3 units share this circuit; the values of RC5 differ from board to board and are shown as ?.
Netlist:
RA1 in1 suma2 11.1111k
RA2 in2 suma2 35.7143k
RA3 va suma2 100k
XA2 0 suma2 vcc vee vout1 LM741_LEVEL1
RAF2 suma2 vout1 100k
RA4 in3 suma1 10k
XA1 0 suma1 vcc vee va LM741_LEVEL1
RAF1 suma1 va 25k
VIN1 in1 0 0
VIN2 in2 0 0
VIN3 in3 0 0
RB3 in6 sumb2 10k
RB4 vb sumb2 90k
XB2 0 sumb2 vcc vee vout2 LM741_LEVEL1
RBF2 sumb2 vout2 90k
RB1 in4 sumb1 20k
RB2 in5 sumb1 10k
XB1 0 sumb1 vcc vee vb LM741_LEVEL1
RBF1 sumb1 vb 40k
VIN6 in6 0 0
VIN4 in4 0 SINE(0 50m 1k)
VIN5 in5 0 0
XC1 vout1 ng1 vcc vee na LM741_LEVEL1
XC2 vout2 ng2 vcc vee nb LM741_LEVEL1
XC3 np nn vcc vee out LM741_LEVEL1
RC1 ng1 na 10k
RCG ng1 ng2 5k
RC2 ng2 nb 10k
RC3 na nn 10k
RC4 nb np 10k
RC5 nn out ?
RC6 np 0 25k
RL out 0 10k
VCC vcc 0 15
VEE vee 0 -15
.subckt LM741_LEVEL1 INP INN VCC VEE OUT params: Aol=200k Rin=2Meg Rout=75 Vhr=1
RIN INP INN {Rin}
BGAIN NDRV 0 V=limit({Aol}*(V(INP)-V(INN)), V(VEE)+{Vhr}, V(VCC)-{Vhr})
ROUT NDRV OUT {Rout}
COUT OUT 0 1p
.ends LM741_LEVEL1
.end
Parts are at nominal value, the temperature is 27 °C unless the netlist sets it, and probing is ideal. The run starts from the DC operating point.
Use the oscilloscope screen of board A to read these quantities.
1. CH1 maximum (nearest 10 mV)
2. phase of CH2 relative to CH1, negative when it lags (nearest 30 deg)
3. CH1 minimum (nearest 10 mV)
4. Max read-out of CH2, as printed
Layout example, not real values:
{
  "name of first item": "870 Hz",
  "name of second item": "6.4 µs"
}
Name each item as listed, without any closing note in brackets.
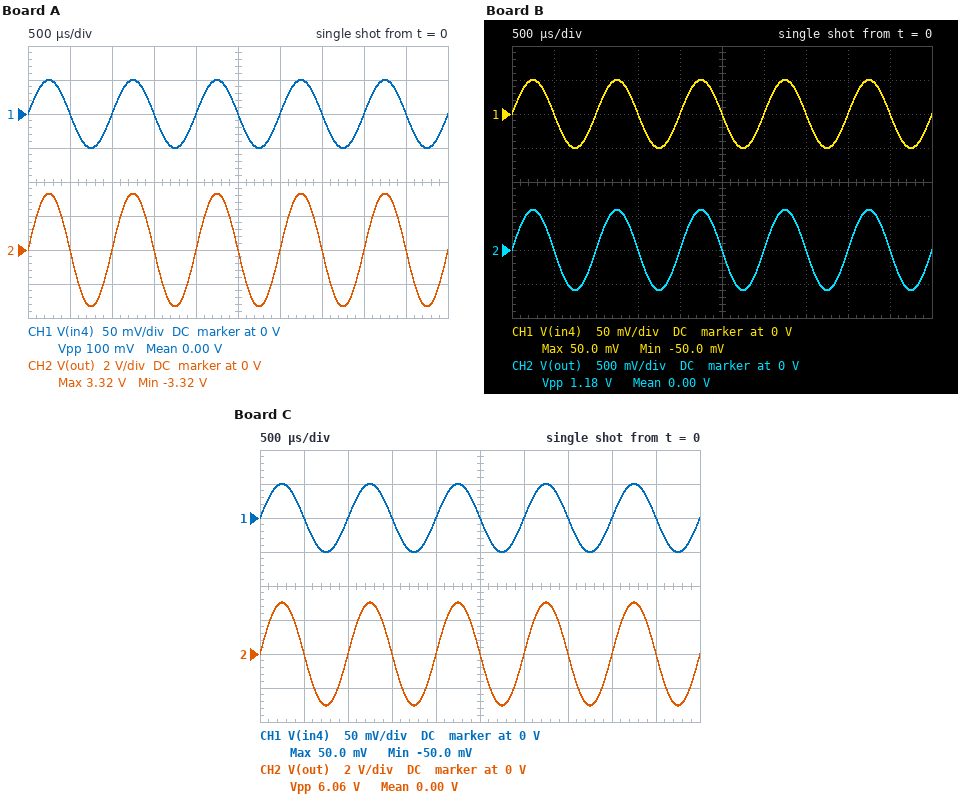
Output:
{
  "CH1 maximum": "50 mV",
  "phase of CH2 relative to CH1, negative when it lags": "0 deg",
  "CH1 minimum": "-50 mV",
  "Max read-out of CH2, as printed": "3.32 V"
}
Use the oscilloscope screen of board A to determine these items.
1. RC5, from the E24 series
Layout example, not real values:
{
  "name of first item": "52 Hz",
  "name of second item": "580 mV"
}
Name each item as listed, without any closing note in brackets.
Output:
{
  "RC5, from the E24 series": "75 kΩ"
}
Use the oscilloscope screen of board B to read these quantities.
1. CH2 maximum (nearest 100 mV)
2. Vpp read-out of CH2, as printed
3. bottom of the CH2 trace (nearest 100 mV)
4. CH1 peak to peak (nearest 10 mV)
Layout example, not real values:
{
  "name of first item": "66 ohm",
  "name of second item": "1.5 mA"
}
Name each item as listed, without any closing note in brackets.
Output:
{
  "CH2 maximum": "600 mV",
  "Vpp read-out of CH2, as printed": "1.18 V",
  "bottom of the CH2 trace": "-600 mV",
  "CH1 peak to peak": "100 mV"
}
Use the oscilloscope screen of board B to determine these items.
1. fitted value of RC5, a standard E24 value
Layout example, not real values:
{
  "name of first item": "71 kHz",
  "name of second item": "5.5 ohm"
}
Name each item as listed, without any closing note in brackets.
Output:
{
  "fitted value of RC5, a standard E24 value": "9.1 kΩ"
}
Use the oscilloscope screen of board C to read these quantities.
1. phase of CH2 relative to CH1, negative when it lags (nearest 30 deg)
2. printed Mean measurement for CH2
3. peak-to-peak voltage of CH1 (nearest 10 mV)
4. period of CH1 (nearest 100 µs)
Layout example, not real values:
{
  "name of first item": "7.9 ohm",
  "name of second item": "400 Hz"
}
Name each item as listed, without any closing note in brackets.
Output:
{
  "phase of CH2 relative to CH1, negative when it lags": "0 deg",
  "printed Mean measurement for CH2": "0.00 V",
  "peak-to-peak voltage of CH1": "100 mV",
  "period of CH1": "1.0 ms"
}
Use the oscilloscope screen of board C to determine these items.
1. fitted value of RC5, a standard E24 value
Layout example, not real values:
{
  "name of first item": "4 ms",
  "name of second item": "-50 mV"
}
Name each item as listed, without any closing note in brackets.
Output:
{
  "fitted value of RC5, a standard E24 value": "68 kΩ"
}
